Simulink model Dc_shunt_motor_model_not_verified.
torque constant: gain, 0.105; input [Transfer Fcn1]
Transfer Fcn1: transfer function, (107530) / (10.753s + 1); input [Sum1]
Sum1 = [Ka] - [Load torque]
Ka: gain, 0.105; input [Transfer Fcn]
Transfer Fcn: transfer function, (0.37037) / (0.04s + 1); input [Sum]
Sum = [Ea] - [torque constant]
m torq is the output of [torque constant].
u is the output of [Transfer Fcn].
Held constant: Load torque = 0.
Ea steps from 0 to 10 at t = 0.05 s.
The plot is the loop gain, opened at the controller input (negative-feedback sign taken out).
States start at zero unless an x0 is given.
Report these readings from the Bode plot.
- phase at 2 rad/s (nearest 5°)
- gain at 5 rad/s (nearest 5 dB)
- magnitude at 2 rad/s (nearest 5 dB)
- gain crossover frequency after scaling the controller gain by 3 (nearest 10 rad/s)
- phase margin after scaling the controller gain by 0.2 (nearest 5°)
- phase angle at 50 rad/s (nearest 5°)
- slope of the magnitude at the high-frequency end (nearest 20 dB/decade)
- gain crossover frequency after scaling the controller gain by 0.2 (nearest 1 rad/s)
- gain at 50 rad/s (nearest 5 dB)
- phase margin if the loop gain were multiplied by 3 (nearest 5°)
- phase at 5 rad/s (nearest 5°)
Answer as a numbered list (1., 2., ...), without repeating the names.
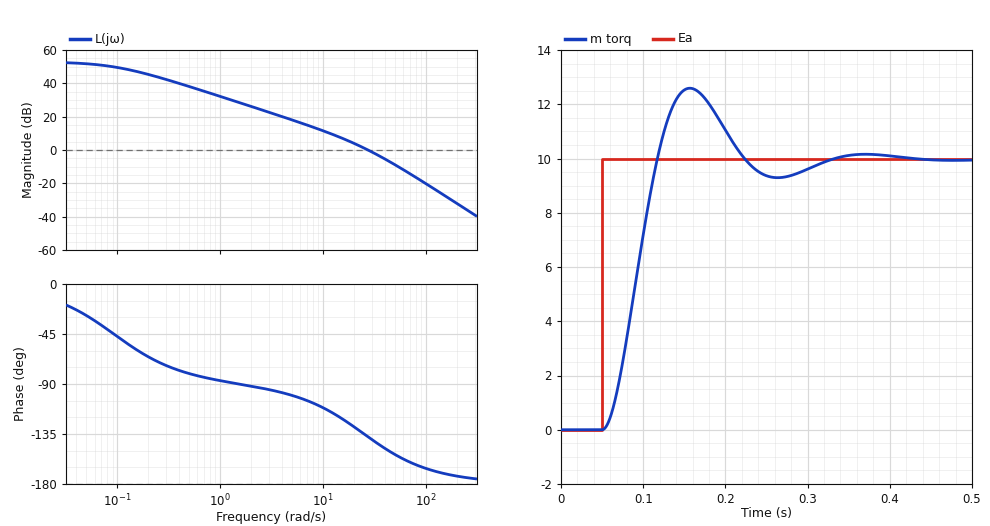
1. -90°
2. 20 dB
3. 25 dB
4. 50 rad/s
5. 75°
6. -155°
7. -40 dB/decade
8. 8 rad/s
9. -10 dB
10. 25°
11. -100°
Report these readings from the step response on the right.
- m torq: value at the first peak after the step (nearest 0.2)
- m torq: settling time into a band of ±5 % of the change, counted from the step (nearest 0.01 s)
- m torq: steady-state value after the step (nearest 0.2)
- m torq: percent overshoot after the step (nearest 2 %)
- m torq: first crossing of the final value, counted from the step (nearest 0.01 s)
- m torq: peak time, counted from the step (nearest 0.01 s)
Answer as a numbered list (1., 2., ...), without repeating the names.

1. 12.6
2. 0.24 s
3. 10.0
4. 26 %
5. 0.07 s
6. 0.11 s
